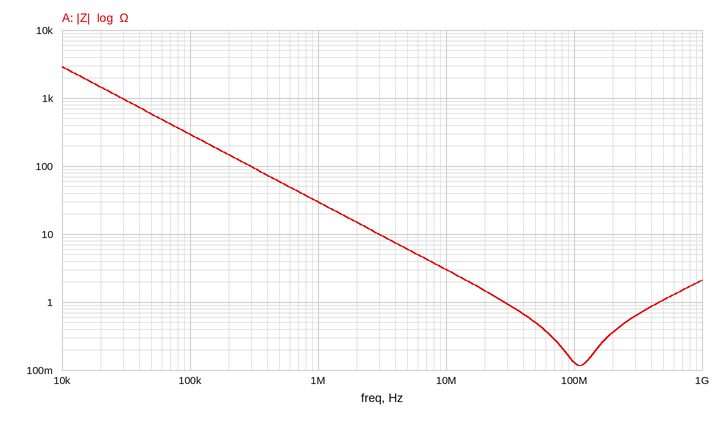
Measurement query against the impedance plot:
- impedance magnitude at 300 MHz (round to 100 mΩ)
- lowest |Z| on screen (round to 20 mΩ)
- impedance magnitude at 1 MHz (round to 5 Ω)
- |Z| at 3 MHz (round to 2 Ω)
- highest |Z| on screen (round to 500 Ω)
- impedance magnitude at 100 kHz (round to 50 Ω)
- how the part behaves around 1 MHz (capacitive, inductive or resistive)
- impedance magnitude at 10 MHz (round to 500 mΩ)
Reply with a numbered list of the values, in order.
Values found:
1. 600 mΩ
2. 120 mΩ
3. 30 Ω
4. 10 Ω
5. 3.0 kΩ
6. 300 Ω
7. capacitive
8. 3.0 Ω
